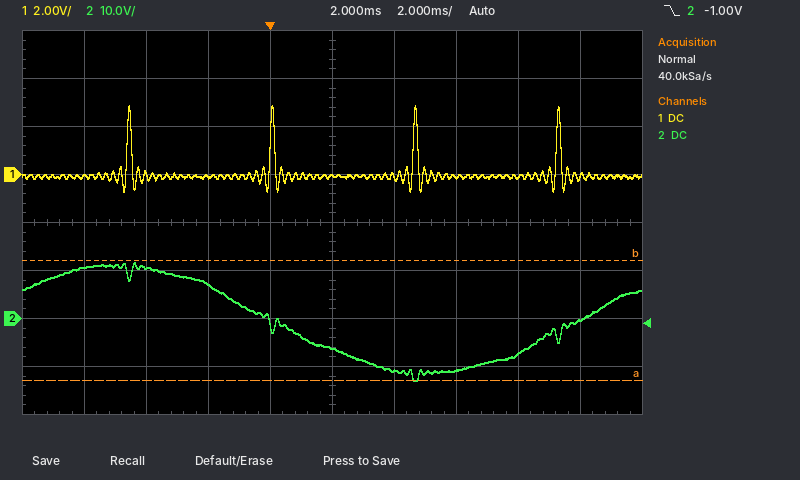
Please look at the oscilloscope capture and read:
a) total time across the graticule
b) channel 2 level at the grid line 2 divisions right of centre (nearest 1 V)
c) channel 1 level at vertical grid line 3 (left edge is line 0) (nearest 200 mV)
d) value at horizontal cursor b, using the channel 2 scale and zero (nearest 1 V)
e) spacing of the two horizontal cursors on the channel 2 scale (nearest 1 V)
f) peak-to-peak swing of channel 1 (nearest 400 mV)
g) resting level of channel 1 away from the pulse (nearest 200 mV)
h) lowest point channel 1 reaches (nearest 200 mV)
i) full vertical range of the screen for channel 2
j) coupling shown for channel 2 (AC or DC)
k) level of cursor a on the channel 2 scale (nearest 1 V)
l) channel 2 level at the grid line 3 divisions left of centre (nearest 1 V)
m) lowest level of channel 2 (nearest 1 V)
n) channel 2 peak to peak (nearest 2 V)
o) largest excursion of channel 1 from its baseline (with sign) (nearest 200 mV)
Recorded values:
20 ms
-11 V
0.0 V
12 V
25 V
3.6 V
0.0 V
-800 mV
80 V
DC
-13 V
11 V
-13 V
24 V
+3.0 V
